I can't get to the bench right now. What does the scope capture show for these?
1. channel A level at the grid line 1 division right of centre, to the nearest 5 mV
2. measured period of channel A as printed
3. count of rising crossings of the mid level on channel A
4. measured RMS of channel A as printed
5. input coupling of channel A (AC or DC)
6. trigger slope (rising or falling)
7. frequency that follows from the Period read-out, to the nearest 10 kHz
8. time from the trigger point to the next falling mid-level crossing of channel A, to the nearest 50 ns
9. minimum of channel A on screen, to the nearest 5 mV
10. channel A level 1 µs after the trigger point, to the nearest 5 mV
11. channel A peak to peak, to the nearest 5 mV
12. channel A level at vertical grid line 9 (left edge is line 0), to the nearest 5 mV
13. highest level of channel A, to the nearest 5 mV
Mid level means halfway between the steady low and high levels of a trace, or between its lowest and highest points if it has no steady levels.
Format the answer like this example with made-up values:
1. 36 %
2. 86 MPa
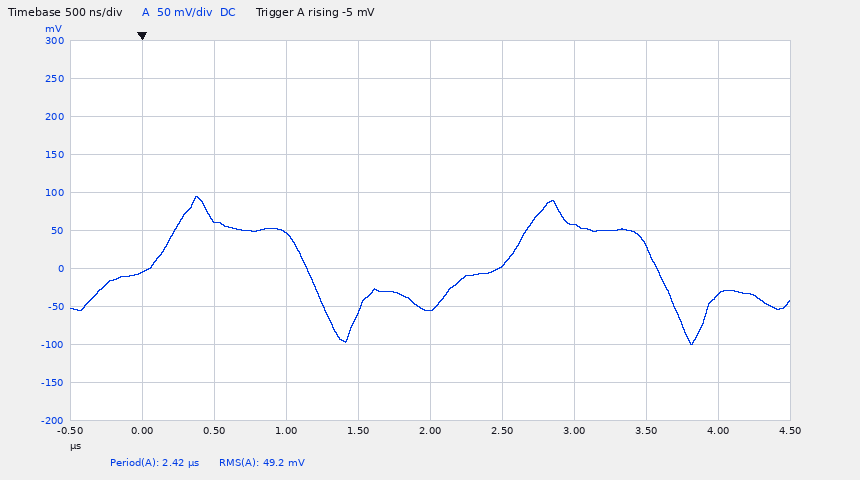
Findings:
1. 5 mV
2. 2.42 µs
3. 2
4. 49.2 mV
5. DC
6. rising
7. 410 kHz
8. 1.15 µs
9. -100 mV
10. 45 mV
11. 195 mV
12. -35 mV
13. 95 mV
